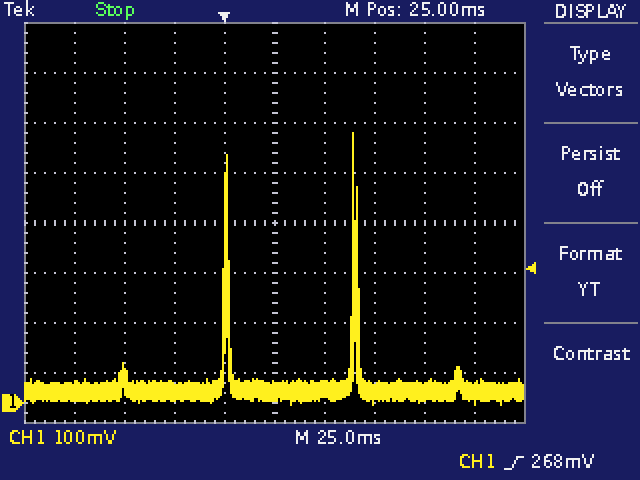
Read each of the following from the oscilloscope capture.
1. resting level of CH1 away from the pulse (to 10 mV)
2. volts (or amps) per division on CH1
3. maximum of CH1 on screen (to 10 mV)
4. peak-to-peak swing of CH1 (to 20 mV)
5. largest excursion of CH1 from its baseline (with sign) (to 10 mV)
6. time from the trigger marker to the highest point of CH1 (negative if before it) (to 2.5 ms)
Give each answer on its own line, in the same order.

20 mV
100 mV
540 mV
540 mV
+520 mV
+65.0 ms
